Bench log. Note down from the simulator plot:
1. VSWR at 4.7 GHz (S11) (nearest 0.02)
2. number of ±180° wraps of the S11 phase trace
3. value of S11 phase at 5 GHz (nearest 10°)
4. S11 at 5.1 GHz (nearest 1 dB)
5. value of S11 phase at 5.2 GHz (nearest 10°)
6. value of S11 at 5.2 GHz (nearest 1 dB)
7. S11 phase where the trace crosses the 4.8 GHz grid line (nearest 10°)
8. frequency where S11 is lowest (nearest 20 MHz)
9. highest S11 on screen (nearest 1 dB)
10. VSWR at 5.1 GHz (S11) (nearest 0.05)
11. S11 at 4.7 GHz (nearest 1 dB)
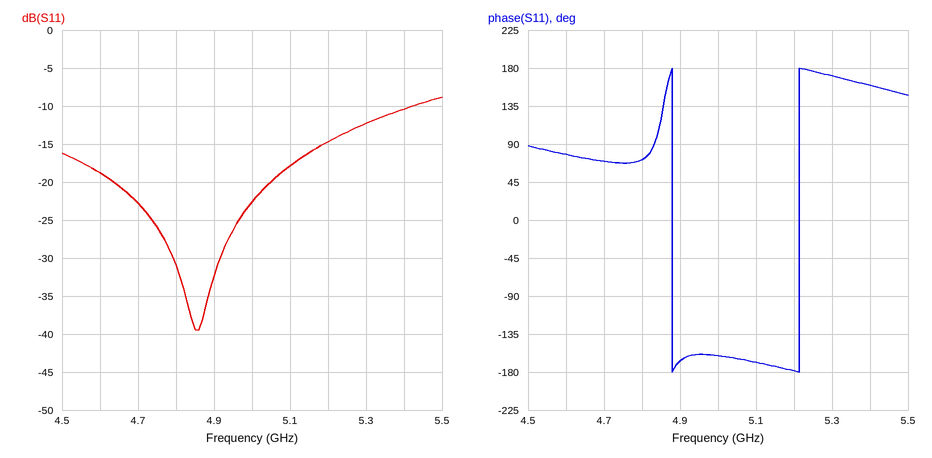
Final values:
1.16
2
-160°
-18 dB
-180°
-15 dB
70°
4.86 GHz
-9 dB
1.30
-23 dB
